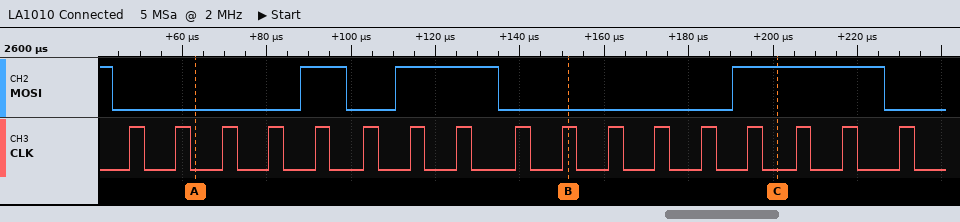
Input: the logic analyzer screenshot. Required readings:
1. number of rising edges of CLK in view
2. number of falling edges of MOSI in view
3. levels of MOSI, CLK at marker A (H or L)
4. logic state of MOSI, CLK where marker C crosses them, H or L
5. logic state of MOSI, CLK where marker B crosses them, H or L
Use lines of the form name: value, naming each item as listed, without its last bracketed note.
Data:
number of rising edges of CLK in view: 17
number of falling edges of MOSI in view: 4
levels of MOSI, CLK at marker A: MOSI=L, CLK=L
logic state of MOSI, CLK where marker C crosses them, H or L: MOSI=H, CLK=L
logic state of MOSI, CLK where marker B crosses them, H or L: MOSI=L, CLK=H
